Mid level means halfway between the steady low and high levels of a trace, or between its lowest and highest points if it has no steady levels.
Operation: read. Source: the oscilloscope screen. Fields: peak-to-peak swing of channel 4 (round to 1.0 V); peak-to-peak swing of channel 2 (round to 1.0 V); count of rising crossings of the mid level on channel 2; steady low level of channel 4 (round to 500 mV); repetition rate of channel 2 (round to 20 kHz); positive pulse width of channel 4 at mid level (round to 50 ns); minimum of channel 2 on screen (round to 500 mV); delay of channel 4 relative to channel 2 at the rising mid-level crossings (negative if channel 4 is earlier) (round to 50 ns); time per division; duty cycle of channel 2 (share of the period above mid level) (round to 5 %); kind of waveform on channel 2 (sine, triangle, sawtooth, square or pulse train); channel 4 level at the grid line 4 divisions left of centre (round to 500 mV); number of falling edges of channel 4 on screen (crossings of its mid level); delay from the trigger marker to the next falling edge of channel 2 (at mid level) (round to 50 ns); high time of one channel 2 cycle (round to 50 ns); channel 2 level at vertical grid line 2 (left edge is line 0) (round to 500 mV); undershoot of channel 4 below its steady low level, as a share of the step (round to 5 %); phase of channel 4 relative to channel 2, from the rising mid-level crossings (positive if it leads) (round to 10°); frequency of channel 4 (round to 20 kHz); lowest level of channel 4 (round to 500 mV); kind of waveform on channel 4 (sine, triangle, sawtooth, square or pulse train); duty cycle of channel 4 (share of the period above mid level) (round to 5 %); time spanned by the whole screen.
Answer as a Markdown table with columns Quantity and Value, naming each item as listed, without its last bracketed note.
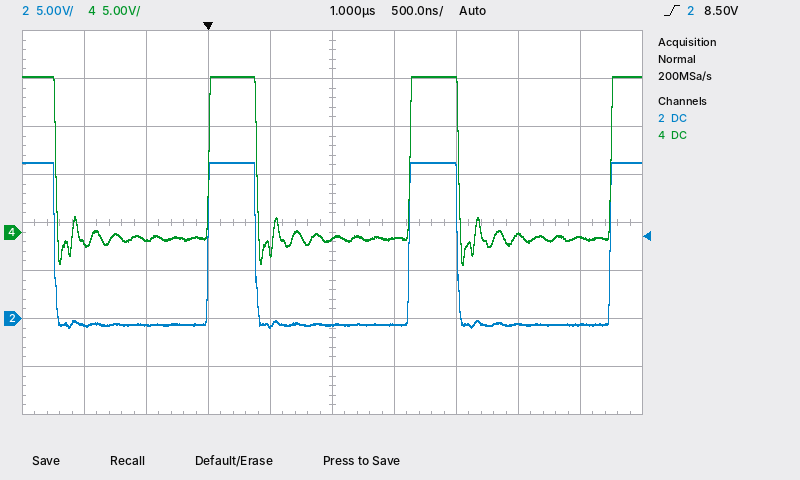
| Quantity | Value |
|---|---|
| peak-to-peak swing of channel 4 | 20.0 V |
| peak-to-peak swing of channel 2 | 17.0 V |
| count of rising crossings of the mid level on channel 2 | 3 |
| steady low level of channel 4 | -500 mV |
| repetition rate of channel 2 | 620 kHz |
| positive pulse width of channel 4 at mid level | 400 ns |
| minimum of channel 2 on screen | -1.0 V |
| delay of channel 4 relative to channel 2 at the rising mid-level crossings (negative if channel 4 is earlier) | 0 ns |
| time per division | 500 ns |
| duty cycle of channel 2 (share of the period above mid level) | 25 % |
| kind of waveform on channel 2 | pulse train |
| channel 4 level at the grid line 4 divisions left of centre | -1.0 V |
| number of falling edges of channel 4 on screen | 3 |
| delay from the trigger marker to the next falling edge of channel 2 (at mid level) | 400 ns |
| high time of one channel 2 cycle | 400 ns |
| channel 2 level at vertical grid line 2 (left edge is line 0) | -500 mV |
| undershoot of channel 4 below its steady low level, as a share of the step | 15 % |
| phase of channel 4 relative to channel 2, from the rising mid-level crossings (positive if it leads) | 0° |
| frequency of channel 4 | 620 kHz |
| lowest level of channel 4 | -3.5 V |
| kind of waveform on channel 4 | pulse train |
| duty cycle of channel 4 (share of the period above mid level) | 25 % |
| time spanned by the whole screen | 5 µs |
